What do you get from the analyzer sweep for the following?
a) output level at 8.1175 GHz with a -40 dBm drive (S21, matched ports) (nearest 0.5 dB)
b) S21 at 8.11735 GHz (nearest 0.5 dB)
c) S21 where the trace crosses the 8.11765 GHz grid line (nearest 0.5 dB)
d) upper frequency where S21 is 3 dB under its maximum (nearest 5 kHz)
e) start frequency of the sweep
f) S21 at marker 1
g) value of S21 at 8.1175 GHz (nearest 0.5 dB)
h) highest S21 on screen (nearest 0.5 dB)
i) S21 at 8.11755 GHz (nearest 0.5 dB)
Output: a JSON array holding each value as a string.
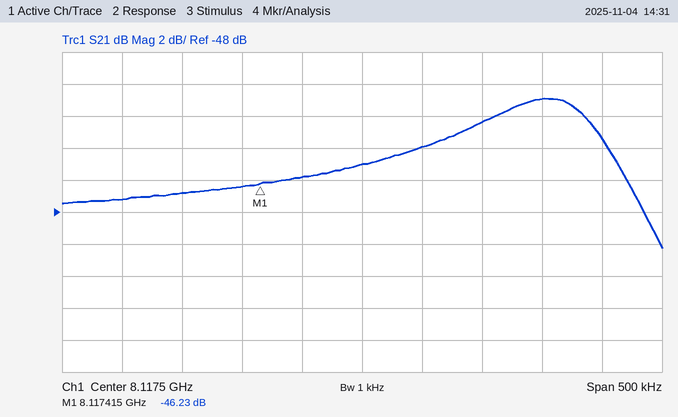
["-85.0 dBm", "-47.0 dB", "-41.0 dB", "8.117705 GHz", "8.11725 GHz", "-46.23 dB", "-45.0 dB", "-41.0 dB", "-44.0 dB"]
